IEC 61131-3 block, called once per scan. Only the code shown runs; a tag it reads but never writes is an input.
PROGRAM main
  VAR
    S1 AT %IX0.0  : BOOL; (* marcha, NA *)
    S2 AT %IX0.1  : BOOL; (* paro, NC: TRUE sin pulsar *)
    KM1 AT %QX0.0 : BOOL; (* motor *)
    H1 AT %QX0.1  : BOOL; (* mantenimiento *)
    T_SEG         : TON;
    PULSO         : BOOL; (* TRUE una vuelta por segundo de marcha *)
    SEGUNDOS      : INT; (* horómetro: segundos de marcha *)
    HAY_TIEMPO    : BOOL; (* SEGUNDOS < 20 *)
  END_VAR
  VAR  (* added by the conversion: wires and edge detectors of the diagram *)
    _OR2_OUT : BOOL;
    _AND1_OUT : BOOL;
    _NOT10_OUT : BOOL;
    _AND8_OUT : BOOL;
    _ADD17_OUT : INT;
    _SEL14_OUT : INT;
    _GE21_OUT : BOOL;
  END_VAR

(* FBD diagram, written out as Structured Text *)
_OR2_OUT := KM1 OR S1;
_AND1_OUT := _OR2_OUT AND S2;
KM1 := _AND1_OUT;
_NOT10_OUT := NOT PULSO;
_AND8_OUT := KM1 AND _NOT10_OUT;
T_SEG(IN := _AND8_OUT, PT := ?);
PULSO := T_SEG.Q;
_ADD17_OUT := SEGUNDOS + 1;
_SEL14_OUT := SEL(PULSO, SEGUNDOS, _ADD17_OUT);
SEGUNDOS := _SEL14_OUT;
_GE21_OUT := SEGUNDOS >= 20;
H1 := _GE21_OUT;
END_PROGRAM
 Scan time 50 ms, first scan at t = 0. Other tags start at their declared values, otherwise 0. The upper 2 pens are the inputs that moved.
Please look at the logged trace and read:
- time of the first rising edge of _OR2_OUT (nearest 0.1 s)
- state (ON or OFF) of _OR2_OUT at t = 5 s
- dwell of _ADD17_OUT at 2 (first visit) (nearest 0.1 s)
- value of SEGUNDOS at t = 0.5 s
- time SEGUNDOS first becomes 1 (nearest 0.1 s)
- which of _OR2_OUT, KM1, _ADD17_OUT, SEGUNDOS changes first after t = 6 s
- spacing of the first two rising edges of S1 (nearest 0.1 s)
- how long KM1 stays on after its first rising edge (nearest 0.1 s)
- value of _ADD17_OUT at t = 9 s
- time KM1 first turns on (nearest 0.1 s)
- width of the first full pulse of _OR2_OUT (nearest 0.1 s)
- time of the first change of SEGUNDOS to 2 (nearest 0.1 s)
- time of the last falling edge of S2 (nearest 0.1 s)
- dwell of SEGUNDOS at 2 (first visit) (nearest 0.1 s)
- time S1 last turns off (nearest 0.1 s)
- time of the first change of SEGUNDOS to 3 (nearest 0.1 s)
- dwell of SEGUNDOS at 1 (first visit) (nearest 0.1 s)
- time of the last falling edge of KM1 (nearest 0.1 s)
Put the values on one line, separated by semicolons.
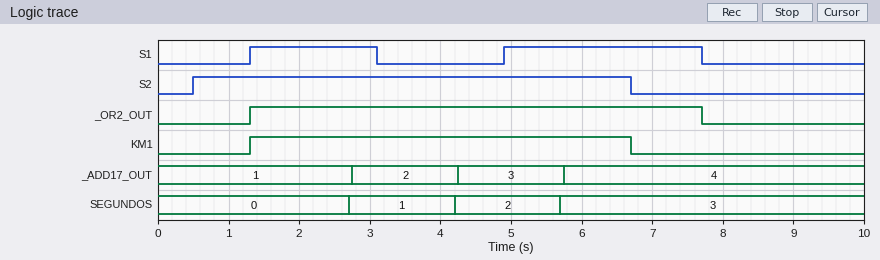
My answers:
1.3 s; ON; 1.5 s; 0; 2.7 s; KM1; 3.6 s; 5.4 s; 4; 1.3 s; 6.4 s; 4.2 s; 6.7 s; 1.5 s; 7.7 s; 5.7 s; 1.5 s; 6.7 s
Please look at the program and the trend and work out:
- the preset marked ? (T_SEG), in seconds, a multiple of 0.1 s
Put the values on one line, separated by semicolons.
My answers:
1.4 s
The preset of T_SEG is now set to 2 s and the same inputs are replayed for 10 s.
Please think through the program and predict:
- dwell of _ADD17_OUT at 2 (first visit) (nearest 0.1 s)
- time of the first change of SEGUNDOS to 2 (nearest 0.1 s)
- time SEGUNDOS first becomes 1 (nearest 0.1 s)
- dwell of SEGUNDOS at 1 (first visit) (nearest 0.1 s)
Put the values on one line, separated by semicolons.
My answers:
2.1 s; 5.4 s; 3.3 s; 2.1 s
